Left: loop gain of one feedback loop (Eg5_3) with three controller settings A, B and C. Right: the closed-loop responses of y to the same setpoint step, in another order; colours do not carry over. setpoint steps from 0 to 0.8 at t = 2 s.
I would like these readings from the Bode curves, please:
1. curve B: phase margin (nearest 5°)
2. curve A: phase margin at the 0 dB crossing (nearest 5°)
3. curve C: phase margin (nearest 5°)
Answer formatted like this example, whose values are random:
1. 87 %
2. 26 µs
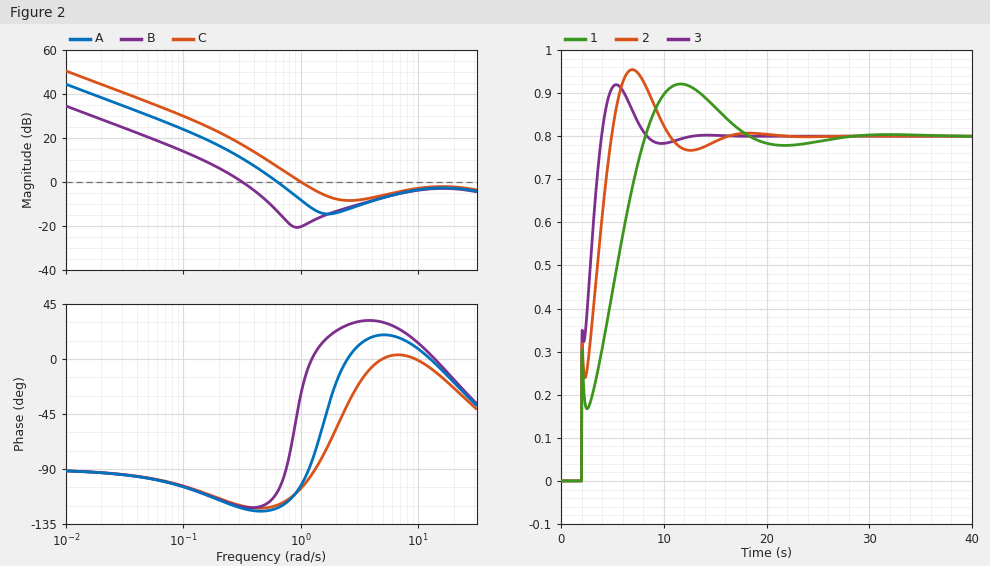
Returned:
1. 60°
2. 60°
3. 75°
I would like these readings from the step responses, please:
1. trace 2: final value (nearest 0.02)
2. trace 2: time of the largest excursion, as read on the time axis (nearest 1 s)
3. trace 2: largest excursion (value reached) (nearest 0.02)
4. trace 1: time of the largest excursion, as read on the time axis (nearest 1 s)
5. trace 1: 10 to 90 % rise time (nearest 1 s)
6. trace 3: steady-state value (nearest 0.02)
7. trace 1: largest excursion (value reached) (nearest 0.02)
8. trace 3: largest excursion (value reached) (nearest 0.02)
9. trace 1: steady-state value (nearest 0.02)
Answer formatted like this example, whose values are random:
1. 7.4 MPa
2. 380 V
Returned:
1. 0.80
2. 7 s
3. 0.96
4. 12 s
5. 5 s
6. 0.80
7. 0.92
8. 0.92
9. 0.80
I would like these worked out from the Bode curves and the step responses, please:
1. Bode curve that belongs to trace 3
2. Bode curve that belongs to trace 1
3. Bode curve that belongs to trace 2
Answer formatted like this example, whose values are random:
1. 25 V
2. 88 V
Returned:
1. C
2. B
3. A
